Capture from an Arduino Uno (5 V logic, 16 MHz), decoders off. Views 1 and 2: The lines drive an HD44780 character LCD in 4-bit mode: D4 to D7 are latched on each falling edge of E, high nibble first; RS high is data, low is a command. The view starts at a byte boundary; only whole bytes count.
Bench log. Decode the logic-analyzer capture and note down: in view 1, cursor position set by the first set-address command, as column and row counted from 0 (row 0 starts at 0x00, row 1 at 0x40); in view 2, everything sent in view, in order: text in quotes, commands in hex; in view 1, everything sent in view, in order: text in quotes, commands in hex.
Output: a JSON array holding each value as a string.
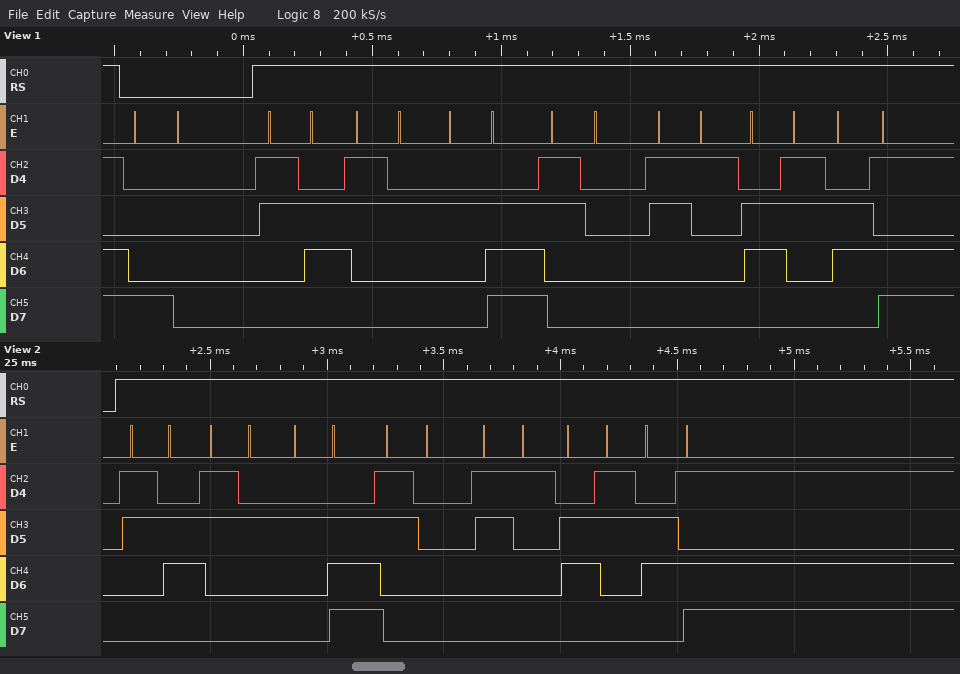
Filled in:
["column 0, row 0", "\"62.01cm\"", "0x80 \"62.01cm\""]
